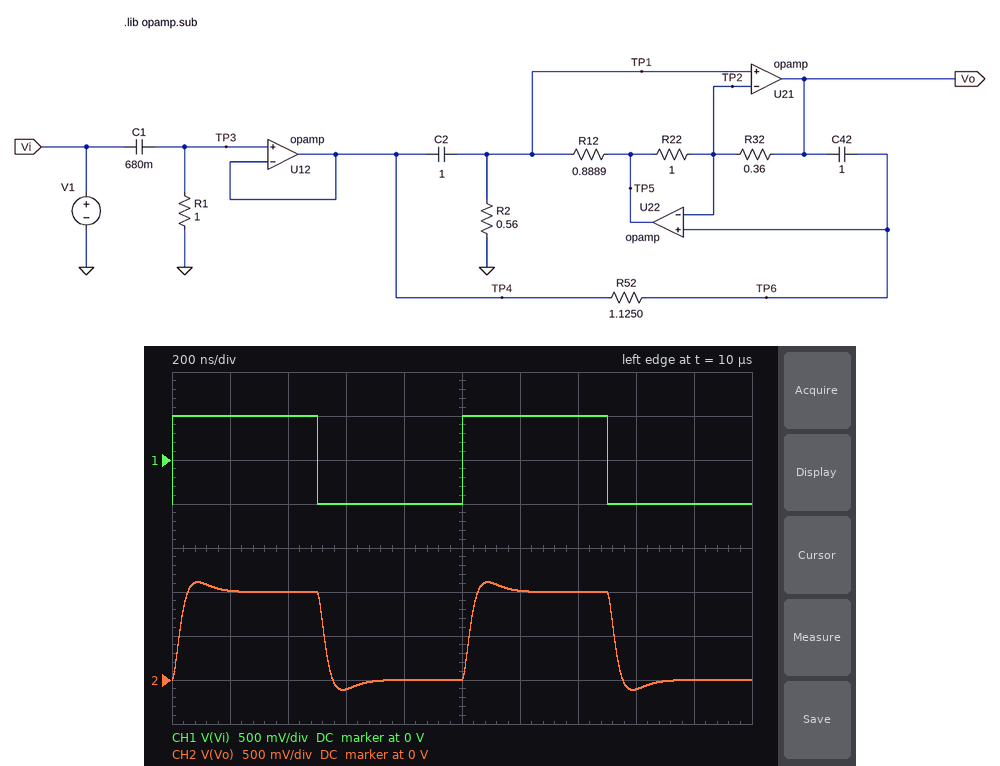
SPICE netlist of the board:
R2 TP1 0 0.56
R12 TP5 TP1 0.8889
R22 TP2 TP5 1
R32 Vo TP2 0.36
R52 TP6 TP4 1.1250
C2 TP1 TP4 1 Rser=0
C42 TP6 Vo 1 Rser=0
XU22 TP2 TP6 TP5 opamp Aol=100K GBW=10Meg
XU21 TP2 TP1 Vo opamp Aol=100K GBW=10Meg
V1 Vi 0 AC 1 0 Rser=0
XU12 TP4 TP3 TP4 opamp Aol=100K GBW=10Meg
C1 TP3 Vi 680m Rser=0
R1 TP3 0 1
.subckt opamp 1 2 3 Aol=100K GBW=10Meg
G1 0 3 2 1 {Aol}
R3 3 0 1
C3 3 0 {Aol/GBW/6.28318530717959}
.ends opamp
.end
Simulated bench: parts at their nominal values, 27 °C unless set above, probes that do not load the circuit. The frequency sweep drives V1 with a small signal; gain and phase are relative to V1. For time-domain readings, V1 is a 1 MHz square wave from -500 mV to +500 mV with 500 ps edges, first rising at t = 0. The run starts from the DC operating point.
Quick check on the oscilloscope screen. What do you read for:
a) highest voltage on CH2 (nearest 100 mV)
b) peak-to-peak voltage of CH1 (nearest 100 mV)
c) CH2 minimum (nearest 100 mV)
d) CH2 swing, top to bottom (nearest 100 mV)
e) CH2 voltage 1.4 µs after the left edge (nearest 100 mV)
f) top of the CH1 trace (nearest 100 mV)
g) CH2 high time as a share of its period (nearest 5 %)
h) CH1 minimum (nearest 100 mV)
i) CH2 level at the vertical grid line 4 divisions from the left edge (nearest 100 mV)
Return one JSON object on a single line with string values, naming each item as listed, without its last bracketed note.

{"highest voltage on CH2": "1.1 V", "peak-to-peak voltage of CH1": "1.0 V", "CH2 minimum": "-100 mV", "CH2 swing, top to bottom": "1.2 V", "CH2 voltage 1.4 µs after the left edge": "1.0 V", "top of the CH1 trace": "500 mV", "CH2 high time as a share of its period": "50 %", "CH1 minimum": "-500 mV", "CH2 level at the vertical grid line 4 divisions from the left edge": "0 V"}
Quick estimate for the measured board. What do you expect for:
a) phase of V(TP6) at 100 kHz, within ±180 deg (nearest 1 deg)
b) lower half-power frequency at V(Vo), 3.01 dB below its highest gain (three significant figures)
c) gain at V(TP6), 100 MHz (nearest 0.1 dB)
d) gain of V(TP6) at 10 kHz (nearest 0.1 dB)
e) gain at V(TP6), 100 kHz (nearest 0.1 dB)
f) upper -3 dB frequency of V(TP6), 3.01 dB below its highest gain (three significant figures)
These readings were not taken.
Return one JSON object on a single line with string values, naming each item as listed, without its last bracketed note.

{"phase of V(TP6) at 100 kHz, within ±180 deg": "-1 deg", "lower half-power frequency at V(Vo), 3.01 dB below its highest gain": "405 mHz", "gain at V(TP6), 100 MHz": "-40.1 dB", "gain of V(TP6) at 10 kHz": "0 dB", "gain at V(TP6), 100 kHz": "0 dB", "upper -3 dB frequency of V(TP6), 3.01 dB below its highest gain": "7.59 MHz"}
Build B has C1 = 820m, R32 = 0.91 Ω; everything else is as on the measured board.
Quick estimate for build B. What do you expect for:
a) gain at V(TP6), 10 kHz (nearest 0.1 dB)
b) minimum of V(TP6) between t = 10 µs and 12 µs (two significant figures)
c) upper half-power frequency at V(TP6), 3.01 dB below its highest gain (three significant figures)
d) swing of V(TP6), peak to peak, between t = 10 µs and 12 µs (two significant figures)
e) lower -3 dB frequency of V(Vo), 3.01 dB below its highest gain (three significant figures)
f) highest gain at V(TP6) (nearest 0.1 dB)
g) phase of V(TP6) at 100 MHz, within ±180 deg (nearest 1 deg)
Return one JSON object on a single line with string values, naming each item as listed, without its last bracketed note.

{"gain at V(TP6), 10 kHz": "0 dB", "minimum of V(TP6) between t = 10 µs and 12 µs": "-140 mV", "upper half-power frequency at V(TP6), 3.01 dB below its highest gain": "8.86 MHz", "swing of V(TP6), peak to peak, between t = 10 µs and 12 µs": "1.3 V", "lower -3 dB frequency of V(Vo), 3.01 dB below its highest gain": "289 mHz", "highest gain at V(TP6)": "1.1 dB", "phase of V(TP6) at 100 MHz, within ±180 deg": "-171 deg"}
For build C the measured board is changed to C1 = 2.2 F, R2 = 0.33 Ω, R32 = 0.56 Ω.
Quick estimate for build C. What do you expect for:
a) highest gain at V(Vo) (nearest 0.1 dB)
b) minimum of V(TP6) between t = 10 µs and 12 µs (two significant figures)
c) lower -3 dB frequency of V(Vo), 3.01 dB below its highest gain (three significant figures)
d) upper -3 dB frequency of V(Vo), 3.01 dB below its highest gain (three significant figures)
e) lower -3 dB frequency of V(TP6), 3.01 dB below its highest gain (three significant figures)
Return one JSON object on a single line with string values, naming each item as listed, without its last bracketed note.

{"highest gain at V(Vo)": "1.0 dB", "minimum of V(TP6) between t = 10 µs and 12 µs": "-130 mV", "lower -3 dB frequency of V(Vo), 3.01 dB below its highest gain": "385 mHz", "upper -3 dB frequency of V(Vo), 3.01 dB below its highest gain": "8.16 MHz", "lower -3 dB frequency of V(TP6), 3.01 dB below its highest gain": "700 mHz"}
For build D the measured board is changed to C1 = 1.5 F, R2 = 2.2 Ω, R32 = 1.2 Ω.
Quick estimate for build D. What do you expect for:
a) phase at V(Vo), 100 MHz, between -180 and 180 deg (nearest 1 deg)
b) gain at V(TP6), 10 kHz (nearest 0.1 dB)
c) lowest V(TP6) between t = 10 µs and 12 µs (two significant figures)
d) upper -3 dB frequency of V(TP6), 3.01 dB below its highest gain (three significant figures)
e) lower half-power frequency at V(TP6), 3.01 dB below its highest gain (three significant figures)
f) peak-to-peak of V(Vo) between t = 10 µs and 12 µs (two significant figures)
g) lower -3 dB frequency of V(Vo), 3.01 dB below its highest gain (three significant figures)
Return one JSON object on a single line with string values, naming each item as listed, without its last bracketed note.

{"phase at V(Vo), 100 MHz, between -180 and 180 deg": "-172 deg", "gain at V(TP6), 10 kHz": "0 dB", "lowest V(TP6) between t = 10 µs and 12 µs": "-150 mV", "upper -3 dB frequency of V(TP6), 3.01 dB below its highest gain": "9.26 MHz", "lower half-power frequency at V(TP6), 3.01 dB below its highest gain": "231 mHz", "peak-to-peak of V(Vo) between t = 10 µs and 12 µs": "1.3 V", "lower -3 dB frequency of V(Vo), 3.01 dB below its highest gain": "146 mHz"}
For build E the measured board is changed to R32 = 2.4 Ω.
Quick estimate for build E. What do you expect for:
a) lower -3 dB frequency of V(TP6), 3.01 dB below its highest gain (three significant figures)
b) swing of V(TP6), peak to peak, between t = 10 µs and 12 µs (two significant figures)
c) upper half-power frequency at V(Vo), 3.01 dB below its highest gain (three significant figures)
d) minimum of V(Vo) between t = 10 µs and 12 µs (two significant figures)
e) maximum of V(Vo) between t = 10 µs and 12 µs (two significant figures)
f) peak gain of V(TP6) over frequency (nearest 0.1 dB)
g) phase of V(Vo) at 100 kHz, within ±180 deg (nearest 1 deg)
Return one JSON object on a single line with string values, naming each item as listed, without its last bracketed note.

{"lower -3 dB frequency of V(TP6), 3.01 dB below its highest gain": "553 mHz", "swing of V(TP6), peak to peak, between t = 10 µs and 12 µs": "1.3 V", "upper half-power frequency at V(Vo), 3.01 dB below its highest gain": "10.2 MHz", "minimum of V(Vo) between t = 10 µs and 12 µs": "-160 mV", "maximum of V(Vo) between t = 10 µs and 12 µs": "1.2 V", "peak gain of V(TP6) over frequency": "1.2 dB", "phase of V(Vo) at 100 kHz, within ±180 deg": "-1 deg"}
